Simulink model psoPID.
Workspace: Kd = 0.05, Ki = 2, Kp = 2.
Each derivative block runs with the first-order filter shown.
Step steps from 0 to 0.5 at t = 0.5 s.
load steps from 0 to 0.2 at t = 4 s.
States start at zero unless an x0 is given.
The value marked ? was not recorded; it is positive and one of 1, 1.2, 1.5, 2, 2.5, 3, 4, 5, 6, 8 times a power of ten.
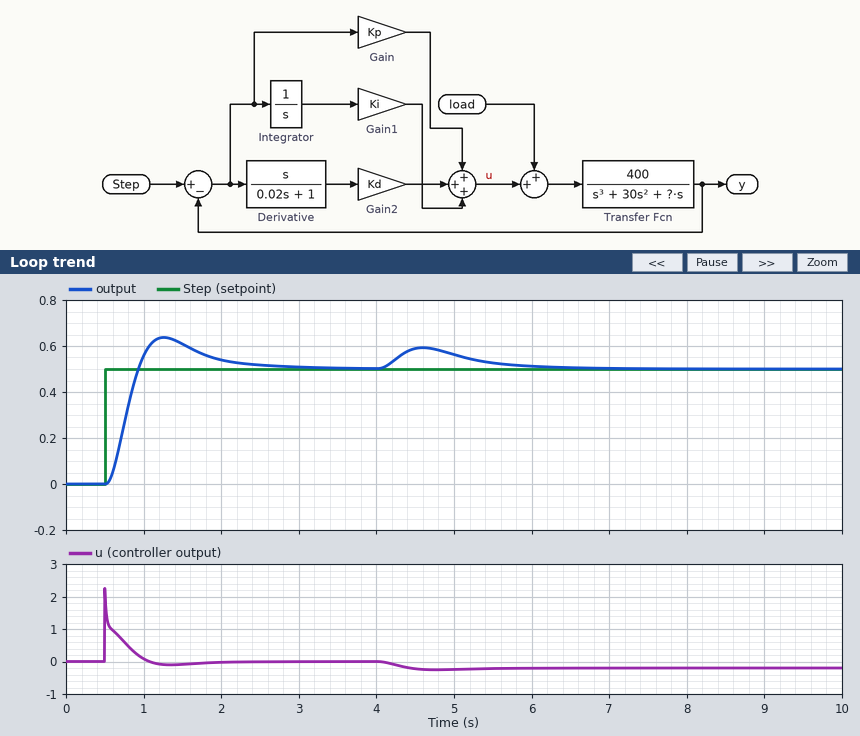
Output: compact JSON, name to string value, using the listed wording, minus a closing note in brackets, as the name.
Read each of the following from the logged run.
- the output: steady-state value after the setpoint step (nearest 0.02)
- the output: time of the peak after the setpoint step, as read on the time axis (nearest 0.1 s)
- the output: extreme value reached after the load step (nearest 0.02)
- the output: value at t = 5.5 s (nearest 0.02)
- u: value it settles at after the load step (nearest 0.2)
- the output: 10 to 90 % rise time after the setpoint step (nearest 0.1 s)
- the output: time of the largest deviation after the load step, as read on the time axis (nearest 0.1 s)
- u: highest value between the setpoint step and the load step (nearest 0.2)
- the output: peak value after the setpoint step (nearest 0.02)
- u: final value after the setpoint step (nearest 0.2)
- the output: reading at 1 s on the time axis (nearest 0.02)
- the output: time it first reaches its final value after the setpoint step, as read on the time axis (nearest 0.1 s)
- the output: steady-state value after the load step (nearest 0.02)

{"the output: steady-state value after the setpoint step": "0.50", "the output: time of the peak after the setpoint step, as read on the time axis": "1.3 s", "the output: extreme value reached after the load step": "0.60", "the output: value at t = 5.5 s": "0.52", "u: value it settles at after the load step": "-0.2", "the output: 10 to 90 % rise time after the setpoint step": "0.3 s", "the output: time of the largest deviation after the load step, as read on the time axis": "4.6 s", "u: highest value between the setpoint step and the load step": "2.2", "the output: peak value after the setpoint step": "0.64", "u: final value after the setpoint step": "0.0", "the output: reading at 1 s on the time axis": "0.56", "the output: time it first reaches its final value after the setpoint step, as read on the time axis": "0.9 s", "the output: steady-state value after the load step": "0.50"}
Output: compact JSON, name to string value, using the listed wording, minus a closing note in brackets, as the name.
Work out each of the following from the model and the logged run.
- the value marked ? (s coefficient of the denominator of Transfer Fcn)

{"the value marked ?": "200"}
